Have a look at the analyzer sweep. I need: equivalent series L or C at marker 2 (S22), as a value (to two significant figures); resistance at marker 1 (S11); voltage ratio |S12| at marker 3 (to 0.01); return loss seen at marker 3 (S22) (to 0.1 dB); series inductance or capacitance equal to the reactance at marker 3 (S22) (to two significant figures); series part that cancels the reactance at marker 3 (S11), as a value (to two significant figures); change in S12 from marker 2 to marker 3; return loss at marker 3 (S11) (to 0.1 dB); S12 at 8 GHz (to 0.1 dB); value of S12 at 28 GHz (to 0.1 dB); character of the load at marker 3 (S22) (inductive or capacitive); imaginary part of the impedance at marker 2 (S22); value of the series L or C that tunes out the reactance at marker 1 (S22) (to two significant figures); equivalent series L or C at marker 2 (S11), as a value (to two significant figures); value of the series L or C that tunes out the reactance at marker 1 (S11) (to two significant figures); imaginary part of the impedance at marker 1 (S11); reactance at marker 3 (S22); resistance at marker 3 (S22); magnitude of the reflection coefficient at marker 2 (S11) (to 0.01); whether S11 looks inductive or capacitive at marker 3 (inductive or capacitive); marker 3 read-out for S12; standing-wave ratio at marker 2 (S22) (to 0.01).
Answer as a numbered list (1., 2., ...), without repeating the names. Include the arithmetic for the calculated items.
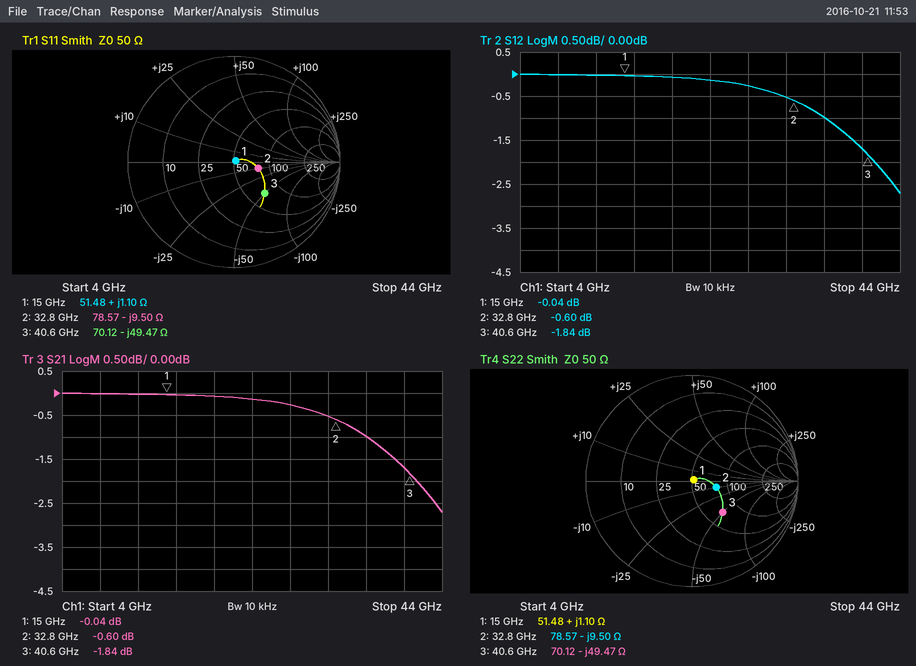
1. C = 1/(2π × 32.8 GHz × 9.5 Ω) ≈ 511 fF, so 510 fF to two significant figures
2. 51.48 Ω
3. 10^(-1.84/20) ≈ 0.81
4. 7.7 dB
5. C = 1/(2π × 40.6 GHz × 49.47 Ω) ≈ 79 fF
6. L = 49.47 Ω/(2π × 40.6 GHz) ≈ 194 pH, so 190 pH to two significant figures
7. -1.84 − (-0.6) = -1.24 dB
8. 7.7 dB
9. 0.0 dB
10. -0.3 dB
11. capacitive
12. -9.50 Ω
13. C = 1/(2π × 15 GHz × 1.1 Ω) ≈ 9.6 pF
14. C = 1/(2π × 32.8 GHz × 9.5 Ω) ≈ 511 fF, so 510 fF to two significant figures
15. C = 1/(2π × 15 GHz × 1.1 Ω) ≈ 9.6 pF
16. +1.10 Ω
17. -49.47 Ω
18. 70.12 Ω
19. 0.23
20. capacitive
21. -1.84 dB
22. 1.61
